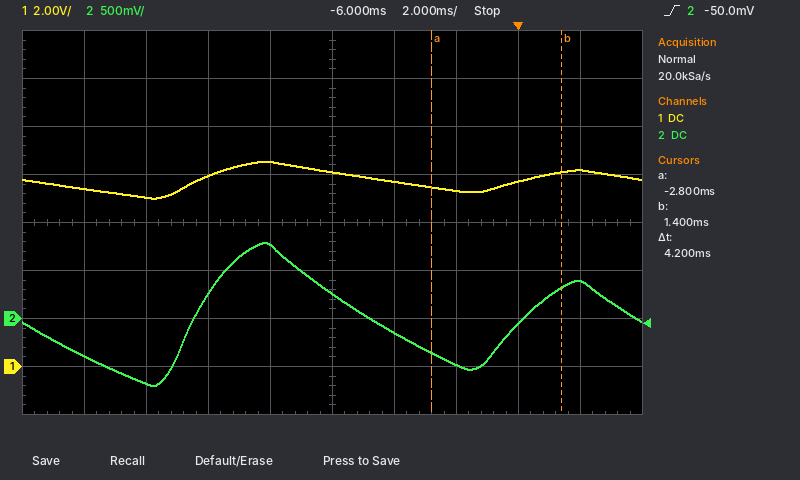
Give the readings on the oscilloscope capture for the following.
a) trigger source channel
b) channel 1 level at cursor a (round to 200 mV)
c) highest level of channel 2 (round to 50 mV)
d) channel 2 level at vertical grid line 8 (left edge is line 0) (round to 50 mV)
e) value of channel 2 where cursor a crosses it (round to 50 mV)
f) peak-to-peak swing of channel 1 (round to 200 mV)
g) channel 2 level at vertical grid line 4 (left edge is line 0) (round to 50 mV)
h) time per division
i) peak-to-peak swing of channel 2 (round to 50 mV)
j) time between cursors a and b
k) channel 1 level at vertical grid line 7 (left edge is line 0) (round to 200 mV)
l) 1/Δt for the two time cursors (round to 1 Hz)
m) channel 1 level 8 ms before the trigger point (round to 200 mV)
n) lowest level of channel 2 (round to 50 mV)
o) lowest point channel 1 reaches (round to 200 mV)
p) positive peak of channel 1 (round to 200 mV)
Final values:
channel 2
7.4 V
800 mV
-50 mV
-350 mV
1.6 V
750 mV
2 ms
1.50 V
4.2 ms
7.4 V
238 Hz
8.6 V
-700 mV
7.0 V
8.6 V
